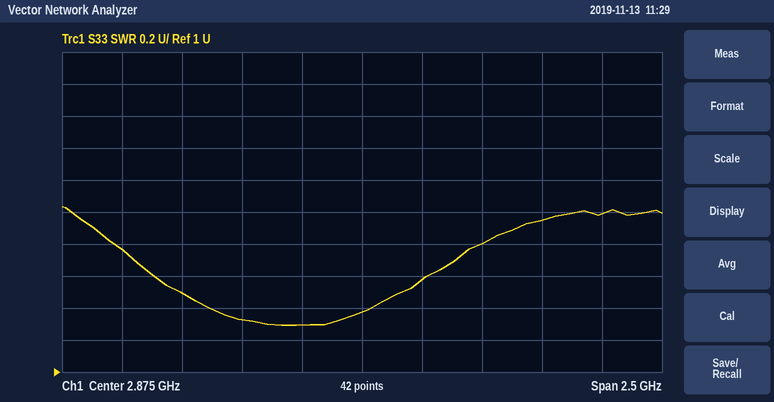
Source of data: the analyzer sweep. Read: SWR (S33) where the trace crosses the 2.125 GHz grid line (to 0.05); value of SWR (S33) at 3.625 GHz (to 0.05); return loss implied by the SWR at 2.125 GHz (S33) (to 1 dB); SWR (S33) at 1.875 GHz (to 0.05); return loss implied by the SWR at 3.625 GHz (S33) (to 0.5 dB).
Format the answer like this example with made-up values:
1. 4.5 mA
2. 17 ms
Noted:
1. 1.50
2. 1.95
3. 14 dB
4. 1.75
5. 10.0 dB
